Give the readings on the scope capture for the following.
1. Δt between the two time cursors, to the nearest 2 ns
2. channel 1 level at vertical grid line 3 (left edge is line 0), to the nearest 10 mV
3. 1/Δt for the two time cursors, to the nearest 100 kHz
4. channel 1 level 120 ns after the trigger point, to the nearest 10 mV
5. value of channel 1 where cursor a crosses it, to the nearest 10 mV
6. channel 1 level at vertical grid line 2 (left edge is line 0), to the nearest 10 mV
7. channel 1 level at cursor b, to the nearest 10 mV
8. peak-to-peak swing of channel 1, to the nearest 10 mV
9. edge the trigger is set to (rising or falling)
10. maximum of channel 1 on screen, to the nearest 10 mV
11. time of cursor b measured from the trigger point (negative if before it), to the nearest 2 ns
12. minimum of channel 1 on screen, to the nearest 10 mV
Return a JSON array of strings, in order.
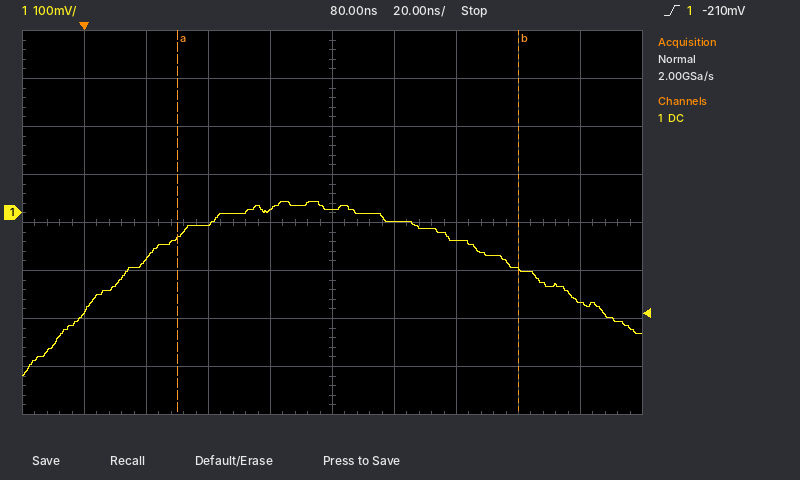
["110 ns", "-20 mV", "9.1 MHz", "-60 mV", "-50 mV", "-100 mV", "-120 mV", "360 mV", "rising", "20 mV", "+140 ns", "-340 mV"]
